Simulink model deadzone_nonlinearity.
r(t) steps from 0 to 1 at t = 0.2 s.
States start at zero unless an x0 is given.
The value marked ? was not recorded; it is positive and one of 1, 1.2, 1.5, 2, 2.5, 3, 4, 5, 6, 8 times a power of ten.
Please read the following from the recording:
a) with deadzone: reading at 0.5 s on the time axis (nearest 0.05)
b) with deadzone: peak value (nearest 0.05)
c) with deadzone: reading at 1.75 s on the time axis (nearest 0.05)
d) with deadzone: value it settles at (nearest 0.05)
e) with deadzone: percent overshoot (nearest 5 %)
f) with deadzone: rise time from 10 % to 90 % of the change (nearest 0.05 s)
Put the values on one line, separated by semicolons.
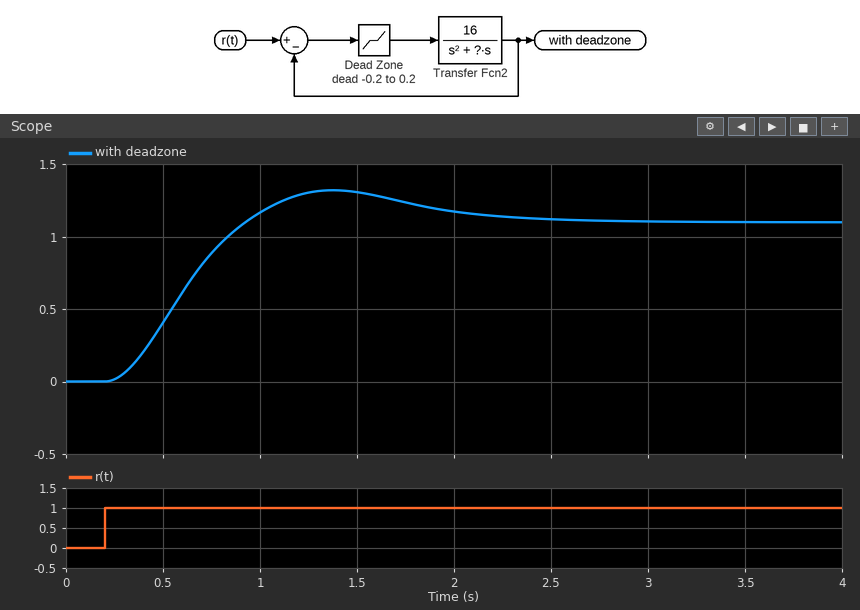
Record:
0.40; 1.30; 1.25; 1.10; 20 %; 0.50 s
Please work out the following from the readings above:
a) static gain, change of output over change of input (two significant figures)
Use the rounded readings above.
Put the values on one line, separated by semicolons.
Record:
1.1
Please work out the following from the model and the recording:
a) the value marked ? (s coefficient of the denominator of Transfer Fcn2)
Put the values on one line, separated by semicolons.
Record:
2.5
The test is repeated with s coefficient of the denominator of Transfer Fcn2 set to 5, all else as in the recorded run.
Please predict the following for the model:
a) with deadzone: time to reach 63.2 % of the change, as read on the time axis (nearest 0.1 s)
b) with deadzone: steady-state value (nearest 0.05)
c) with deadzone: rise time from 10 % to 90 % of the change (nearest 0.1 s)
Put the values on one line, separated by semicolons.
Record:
0.7 s; 0.90; 0.6 s
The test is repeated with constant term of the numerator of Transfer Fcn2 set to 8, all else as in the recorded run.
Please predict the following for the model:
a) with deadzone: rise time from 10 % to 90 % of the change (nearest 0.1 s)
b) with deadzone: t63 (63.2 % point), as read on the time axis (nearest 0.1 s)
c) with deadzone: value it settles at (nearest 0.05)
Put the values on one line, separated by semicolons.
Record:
1.0 s; 0.9 s; 1.15
